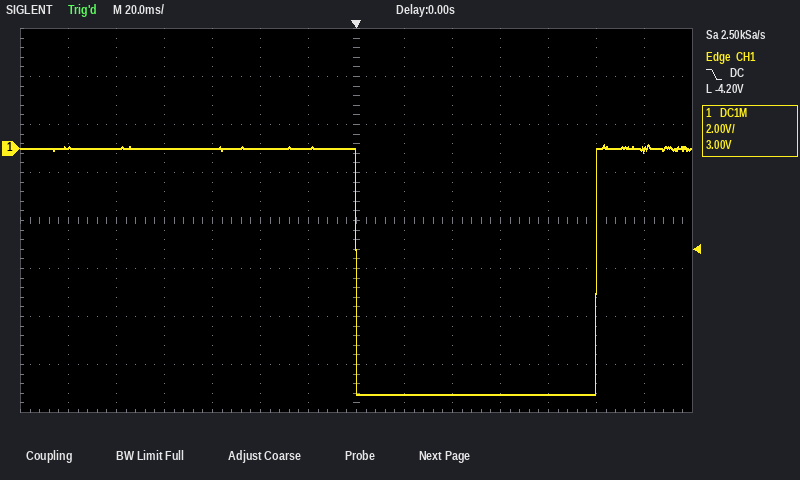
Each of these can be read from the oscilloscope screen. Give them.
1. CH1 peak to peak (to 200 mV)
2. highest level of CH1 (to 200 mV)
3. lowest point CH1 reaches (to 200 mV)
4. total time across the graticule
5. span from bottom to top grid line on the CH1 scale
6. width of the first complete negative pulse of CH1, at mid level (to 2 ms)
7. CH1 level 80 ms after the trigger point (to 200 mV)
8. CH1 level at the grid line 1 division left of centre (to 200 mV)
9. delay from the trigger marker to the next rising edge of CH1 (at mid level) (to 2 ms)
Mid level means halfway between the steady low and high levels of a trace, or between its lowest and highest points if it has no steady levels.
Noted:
10.4 V
200 mV
-10.2 V
280 ms
16 V
100 ms
-10.2 V
0.0 V
100 ms
